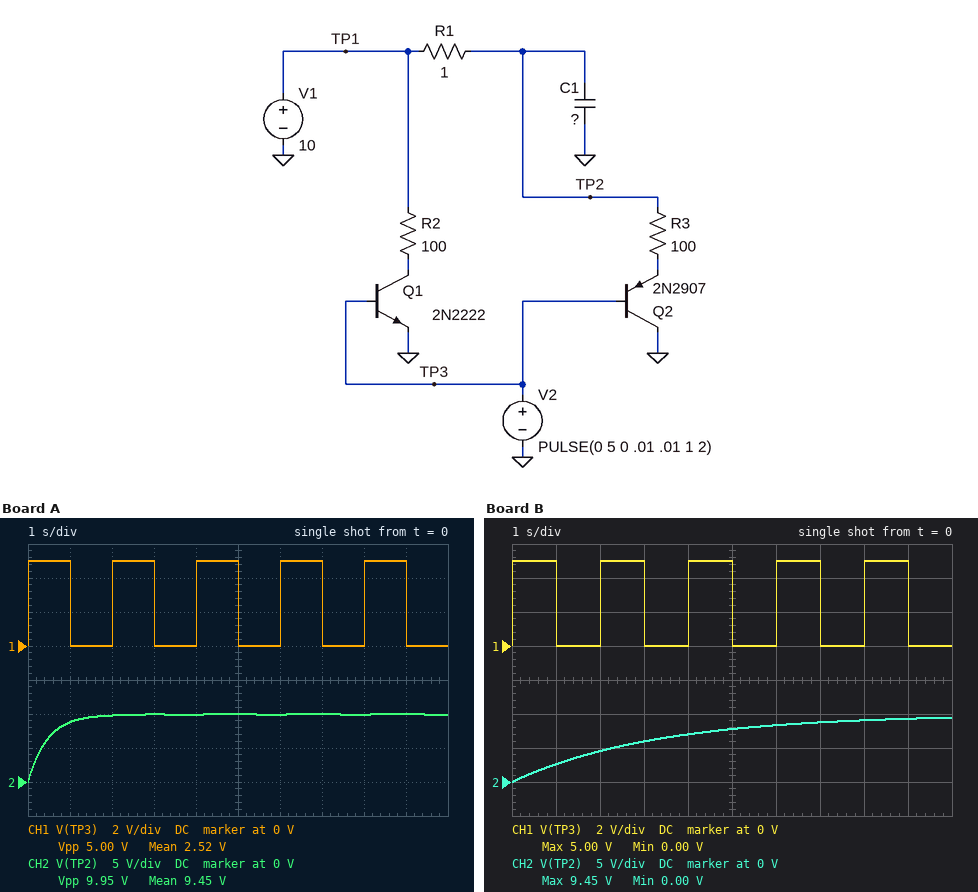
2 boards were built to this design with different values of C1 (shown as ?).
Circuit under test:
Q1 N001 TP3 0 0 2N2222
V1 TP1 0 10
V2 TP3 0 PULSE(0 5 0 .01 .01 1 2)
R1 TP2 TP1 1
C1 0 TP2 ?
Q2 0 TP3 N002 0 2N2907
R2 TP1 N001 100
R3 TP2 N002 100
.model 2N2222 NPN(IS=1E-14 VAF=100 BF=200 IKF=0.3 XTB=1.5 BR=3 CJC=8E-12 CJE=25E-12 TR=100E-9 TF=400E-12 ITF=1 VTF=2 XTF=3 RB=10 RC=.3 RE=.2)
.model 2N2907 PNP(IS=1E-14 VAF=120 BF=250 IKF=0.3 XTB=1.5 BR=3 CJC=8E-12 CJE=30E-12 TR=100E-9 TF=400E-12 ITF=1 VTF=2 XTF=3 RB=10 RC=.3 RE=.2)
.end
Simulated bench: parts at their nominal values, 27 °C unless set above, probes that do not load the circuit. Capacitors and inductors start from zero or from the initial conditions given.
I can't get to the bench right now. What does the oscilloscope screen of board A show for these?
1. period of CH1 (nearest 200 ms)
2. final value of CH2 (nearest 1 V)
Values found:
2.0 s
10 V
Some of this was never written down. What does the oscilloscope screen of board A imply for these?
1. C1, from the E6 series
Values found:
470 mF
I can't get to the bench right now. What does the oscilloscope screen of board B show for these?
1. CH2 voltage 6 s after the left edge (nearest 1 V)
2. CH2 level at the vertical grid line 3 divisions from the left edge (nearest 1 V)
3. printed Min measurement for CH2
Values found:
8 V
6 V
0.00 V
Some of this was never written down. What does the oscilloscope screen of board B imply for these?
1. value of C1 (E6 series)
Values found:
3.3 F
